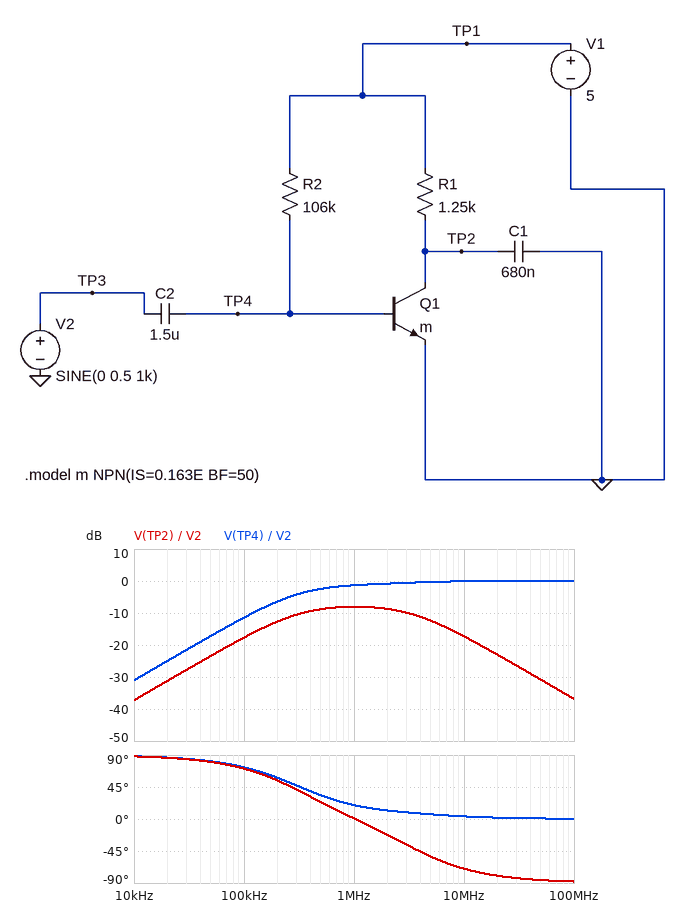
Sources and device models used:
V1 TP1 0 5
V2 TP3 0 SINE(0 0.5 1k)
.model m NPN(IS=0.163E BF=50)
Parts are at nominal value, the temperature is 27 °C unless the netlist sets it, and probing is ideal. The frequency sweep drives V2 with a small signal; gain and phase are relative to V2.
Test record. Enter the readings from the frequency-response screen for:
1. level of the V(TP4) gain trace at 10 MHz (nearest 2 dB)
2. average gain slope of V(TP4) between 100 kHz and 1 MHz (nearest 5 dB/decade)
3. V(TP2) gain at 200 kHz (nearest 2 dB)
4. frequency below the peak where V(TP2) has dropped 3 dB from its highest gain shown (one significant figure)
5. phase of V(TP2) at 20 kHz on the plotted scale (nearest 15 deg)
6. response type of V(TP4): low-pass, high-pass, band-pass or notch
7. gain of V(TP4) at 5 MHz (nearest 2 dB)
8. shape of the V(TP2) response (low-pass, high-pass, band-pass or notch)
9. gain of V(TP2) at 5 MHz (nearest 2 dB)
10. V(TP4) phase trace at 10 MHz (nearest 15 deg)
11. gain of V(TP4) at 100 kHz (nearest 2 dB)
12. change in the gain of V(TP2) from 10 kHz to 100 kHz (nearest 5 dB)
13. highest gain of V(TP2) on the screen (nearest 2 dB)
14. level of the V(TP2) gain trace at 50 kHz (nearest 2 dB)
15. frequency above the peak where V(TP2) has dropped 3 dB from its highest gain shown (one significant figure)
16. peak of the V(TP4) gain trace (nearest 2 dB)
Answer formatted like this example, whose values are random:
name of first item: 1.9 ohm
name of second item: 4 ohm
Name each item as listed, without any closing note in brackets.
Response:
level of the V(TP4) gain trace at 10 MHz: 0 dB
average gain slope of V(TP4) between 100 kHz and 1 MHz: 10 dB/decade
V(TP2) gain at 200 kHz: -12 dB
frequency below the peak where V(TP2) has dropped 3 dB from its highest gain shown: 300 kHz
phase of V(TP2) at 20 kHz on the plotted scale: 90 deg
response type of V(TP4): low-pass, high-pass, band-pass or notch: high-pass
gain of V(TP4) at 5 MHz: 0 dB
shape of the V(TP2) response: band-pass
gain of V(TP2) at 5 MHz: -12 dB
V(TP4) phase trace at 10 MHz: 0 deg
gain of V(TP4) at 100 kHz: -12 dB
change in the gain of V(TP2) from 10 kHz to 100 kHz: 20 dB
highest gain of V(TP2) on the screen: -8 dB
level of the V(TP2) gain trace at 50 kHz: -24 dB
frequency above the peak where V(TP2) has dropped 3 dB from its highest gain shown: 4 MHz
peak of the V(TP4) gain trace: 0 dB
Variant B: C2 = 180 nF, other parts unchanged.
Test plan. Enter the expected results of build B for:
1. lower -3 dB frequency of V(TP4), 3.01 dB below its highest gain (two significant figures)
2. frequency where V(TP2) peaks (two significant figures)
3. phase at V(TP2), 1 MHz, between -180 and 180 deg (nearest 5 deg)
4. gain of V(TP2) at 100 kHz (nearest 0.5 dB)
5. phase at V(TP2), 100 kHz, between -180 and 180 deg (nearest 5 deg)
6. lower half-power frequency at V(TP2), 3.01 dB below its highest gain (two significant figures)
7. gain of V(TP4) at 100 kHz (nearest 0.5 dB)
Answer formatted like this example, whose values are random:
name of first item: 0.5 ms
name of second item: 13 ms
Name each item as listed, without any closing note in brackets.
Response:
lower -3 dB frequency of V(TP4), 3.01 dB below its highest gain: 6.4 MHz
frequency where V(TP2) peaks: 3.0 MHz
phase at V(TP2), 1 MHz, between -180 and 180 deg: 40 deg
gain of V(TP2) at 100 kHz: -35.5 dB
phase at V(TP2), 100 kHz, between -180 and 180 deg: 85 deg
lower half-power frequency at V(TP2), 3.01 dB below its highest gain: 920 kHz
gain of V(TP4) at 100 kHz: -29.5 dB
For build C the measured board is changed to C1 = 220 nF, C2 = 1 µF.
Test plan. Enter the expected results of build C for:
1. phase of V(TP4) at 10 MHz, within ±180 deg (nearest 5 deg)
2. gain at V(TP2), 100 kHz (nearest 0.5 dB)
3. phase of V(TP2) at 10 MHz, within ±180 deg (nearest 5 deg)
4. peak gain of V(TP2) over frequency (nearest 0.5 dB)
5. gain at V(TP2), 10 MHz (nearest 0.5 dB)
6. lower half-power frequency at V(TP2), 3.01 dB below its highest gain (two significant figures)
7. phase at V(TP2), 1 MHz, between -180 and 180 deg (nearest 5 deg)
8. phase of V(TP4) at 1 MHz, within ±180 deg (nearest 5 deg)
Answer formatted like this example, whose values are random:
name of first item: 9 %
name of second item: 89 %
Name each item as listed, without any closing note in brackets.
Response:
phase of V(TP4) at 10 MHz, within ±180 deg: 5 deg
gain at V(TP2), 100 kHz: -21.0 dB
phase of V(TP2) at 10 MHz, within ±180 deg: -45 deg
peak gain of V(TP2) over frequency: -7.0 dB
gain at V(TP2), 10 MHz: -10.0 dB
lower half-power frequency at V(TP2), 3.01 dB below its highest gain: 460 kHz
phase at V(TP2), 1 MHz, between -180 and 180 deg: 20 deg
phase of V(TP4) at 1 MHz, within ±180 deg: 25 deg
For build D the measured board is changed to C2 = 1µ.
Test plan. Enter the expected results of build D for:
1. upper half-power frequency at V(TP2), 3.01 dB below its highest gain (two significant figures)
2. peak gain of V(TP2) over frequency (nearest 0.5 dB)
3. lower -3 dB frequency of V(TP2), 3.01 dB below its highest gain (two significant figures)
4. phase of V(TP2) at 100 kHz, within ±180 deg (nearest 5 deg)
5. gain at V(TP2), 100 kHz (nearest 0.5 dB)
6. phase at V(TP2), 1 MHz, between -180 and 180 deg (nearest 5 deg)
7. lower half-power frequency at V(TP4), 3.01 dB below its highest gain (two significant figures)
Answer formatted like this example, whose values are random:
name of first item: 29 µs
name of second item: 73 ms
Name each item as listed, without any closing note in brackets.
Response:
upper half-power frequency at V(TP2), 3.01 dB below its highest gain: 4.3 MHz
peak gain of V(TP2) over frequency: -9.0 dB
lower -3 dB frequency of V(TP2), 3.01 dB below its highest gain: 360 kHz
phase of V(TP2) at 100 kHz, within ±180 deg: 75 deg
gain at V(TP2), 100 kHz: -21.0 dB
phase at V(TP2), 1 MHz, between -180 and 180 deg: 10 deg
lower half-power frequency at V(TP4), 3.01 dB below its highest gain: 690 kHz
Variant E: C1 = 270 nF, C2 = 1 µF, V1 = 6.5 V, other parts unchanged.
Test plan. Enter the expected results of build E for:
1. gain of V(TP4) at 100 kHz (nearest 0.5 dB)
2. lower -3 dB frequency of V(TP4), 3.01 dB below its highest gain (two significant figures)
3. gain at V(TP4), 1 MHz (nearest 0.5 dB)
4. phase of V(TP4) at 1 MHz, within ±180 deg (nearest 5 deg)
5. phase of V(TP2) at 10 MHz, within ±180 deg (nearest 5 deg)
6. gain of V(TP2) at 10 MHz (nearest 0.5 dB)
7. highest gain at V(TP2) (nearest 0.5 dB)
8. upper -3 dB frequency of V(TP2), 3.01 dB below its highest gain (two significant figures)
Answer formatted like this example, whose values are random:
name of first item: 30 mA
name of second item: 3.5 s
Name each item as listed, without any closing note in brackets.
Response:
gain of V(TP4) at 100 kHz: -15.0 dB
lower -3 dB frequency of V(TP4), 3.01 dB below its highest gain: 580 kHz
gain at V(TP4), 1 MHz: -1.5 dB
phase of V(TP4) at 1 MHz, within ±180 deg: 25 deg
phase of V(TP2) at 10 MHz, within ±180 deg: -50 deg
gain of V(TP2) at 10 MHz: -11.0 dB
highest gain at V(TP2): -7.5 dB
upper -3 dB frequency of V(TP2), 3.01 dB below its highest gain: 8.9 MHz
